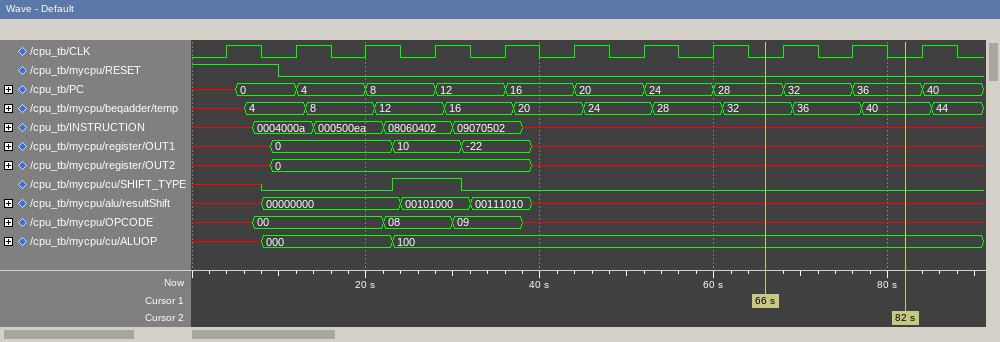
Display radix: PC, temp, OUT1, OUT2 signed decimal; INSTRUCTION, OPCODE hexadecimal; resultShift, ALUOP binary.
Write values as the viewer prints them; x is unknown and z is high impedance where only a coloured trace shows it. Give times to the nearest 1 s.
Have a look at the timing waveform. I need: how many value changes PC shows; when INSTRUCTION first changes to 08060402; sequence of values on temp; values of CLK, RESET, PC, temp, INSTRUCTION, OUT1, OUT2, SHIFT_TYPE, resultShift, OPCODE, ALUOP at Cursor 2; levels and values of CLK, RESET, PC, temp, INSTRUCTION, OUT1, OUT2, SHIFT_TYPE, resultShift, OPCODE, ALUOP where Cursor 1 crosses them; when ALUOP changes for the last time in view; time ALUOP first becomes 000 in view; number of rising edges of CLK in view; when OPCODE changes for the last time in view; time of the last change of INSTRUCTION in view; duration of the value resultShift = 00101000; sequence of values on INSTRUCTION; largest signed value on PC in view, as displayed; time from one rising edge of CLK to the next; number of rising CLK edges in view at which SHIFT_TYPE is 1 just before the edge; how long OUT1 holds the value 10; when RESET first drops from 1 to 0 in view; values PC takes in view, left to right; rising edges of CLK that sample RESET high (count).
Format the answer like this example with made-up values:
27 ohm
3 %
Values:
11
22 s
x, 4, 8, 12, 16, 20, 24, 28, 32, 36, 40, 44
CLK=0, RESET=0, PC=36, temp=40, INSTRUCTION=x, OUT1=x, OUT2=x, SHIFT_TYPE=0, resultShift=x, OPCODE=x, ALUOP=100
CLK=0, RESET=0, PC=28, temp=32, INSTRUCTION=x, OUT1=x, OUT2=x, SHIFT_TYPE=0, resultShift=x, OPCODE=x, ALUOP=100
23 s
8 s
11
38 s
38 s
8 s
x, 0004000a, 000500ea, 08060402, 09070502, x
40
8 s
1
8 s
10 s
x, 0, 4, 8, 12, 16, 20, 24, 28, 32, 36, 40
1
